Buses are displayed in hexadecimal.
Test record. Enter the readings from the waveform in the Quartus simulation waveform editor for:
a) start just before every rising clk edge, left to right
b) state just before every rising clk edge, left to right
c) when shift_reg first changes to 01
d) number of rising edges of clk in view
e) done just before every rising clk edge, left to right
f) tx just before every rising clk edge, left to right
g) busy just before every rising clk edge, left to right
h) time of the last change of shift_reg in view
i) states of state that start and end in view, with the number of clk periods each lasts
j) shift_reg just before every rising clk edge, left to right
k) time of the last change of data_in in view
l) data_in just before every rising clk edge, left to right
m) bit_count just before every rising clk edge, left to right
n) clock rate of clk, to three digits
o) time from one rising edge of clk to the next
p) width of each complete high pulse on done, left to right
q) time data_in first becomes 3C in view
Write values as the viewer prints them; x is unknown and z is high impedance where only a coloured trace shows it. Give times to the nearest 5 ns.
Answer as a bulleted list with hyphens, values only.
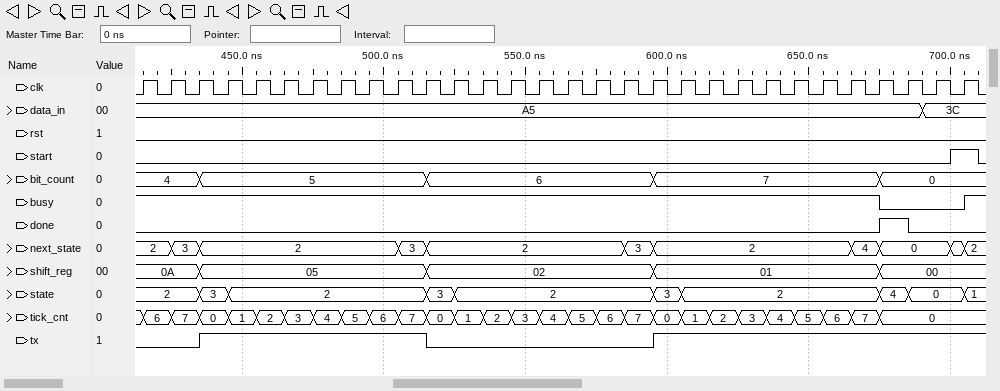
- 0 0 0 0 0 0 0 0 0 0 0 0 0 0 0 0 0 0 0 0 0 0 0 0 0 0 0 0 0 1
- 2, 2, 2, 3, 2, 2, 2, 2, 2, 2, 2, 3, 2, 2, 2, 2, 2, 2, 2, 3, 2, 2, 2, 2, 2, 2, 2, 4, 0, 0
- 595 ns
- 30
- 0 0 0 0 0 0 0 0 0 0 0 0 0 0 0 0 0 0 0 0 0 0 0 0 0 0 0 1 0 0
- 0 0 0 1 1 1 1 1 1 1 1 0 0 0 0 0 0 0 0 1 1 1 1 1 1 1 1 1 1 1
- 1 1 1 1 1 1 1 1 1 1 1 1 1 1 1 1 1 1 1 1 1 1 1 1 1 1 1 0 0 0
- 675 ns
- 3: 1, 2: 7, 3: 1, 2: 7, 3: 1, 2: 7, 4: 1, 0: 2
- 0A, 0A, 0A, 05, 05, 05, 05, 05, 05, 05, 05, 02, 02, 02, 02, 02, 02, 02, 02, 01, 01, 01, 01, 01, 01, 01, 01, 00, 00, 00
- 690 ns
- A5, A5, A5, A5, A5, A5, A5, A5, A5, A5, A5, A5, A5, A5, A5, A5, A5, A5, A5, A5, A5, A5, A5, A5, A5, A5, A5, A5, 3C, 3C
- 4, 4, 4, 5, 5, 5, 5, 5, 5, 5, 5, 6, 6, 6, 6, 6, 6, 6, 6, 7, 7, 7, 7, 7, 7, 7, 7, 0, 0, 0
- 100 MHz
- 10 ns
- 10 ns
- 690 ns
